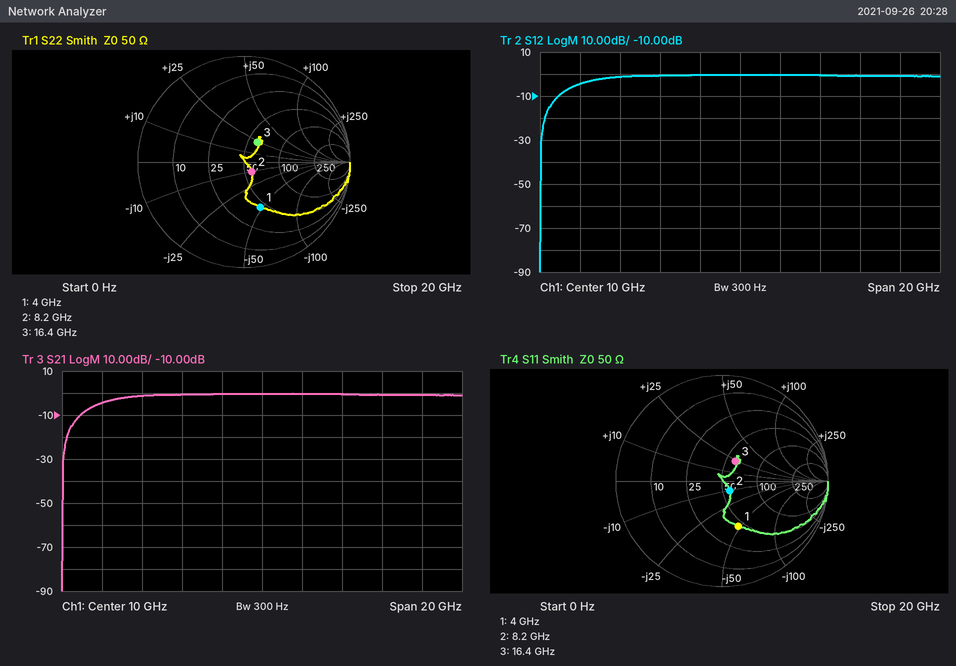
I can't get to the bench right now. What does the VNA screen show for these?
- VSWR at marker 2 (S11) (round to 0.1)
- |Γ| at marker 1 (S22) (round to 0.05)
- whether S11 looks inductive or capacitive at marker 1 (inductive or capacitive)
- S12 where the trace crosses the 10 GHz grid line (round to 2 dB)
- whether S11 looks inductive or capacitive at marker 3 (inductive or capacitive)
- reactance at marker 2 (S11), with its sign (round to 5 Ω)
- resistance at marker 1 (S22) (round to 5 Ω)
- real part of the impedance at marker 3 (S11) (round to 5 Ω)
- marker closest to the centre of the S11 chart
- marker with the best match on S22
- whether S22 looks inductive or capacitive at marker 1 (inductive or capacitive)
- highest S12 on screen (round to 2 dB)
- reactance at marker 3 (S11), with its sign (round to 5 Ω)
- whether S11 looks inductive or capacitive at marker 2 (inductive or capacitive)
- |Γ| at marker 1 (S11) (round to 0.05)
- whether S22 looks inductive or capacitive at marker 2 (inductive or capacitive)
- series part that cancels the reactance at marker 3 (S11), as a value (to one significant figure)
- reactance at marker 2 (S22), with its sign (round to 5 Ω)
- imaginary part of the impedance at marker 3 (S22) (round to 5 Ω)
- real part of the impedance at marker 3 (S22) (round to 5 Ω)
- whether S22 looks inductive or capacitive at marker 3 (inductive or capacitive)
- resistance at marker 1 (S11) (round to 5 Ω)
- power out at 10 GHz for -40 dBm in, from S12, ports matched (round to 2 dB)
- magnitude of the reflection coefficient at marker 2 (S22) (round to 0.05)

1.3
0.45
capacitive
0 dB
inductive
-10 Ω
45 Ω
60 Ω
marker 2
marker 2
capacitive
0 dB
+25 Ω
capacitive
0.45
capacitive
400 fF
-10 Ω
+25 Ω
60 Ω
inductive
45 Ω
-40 dBm
0.10
